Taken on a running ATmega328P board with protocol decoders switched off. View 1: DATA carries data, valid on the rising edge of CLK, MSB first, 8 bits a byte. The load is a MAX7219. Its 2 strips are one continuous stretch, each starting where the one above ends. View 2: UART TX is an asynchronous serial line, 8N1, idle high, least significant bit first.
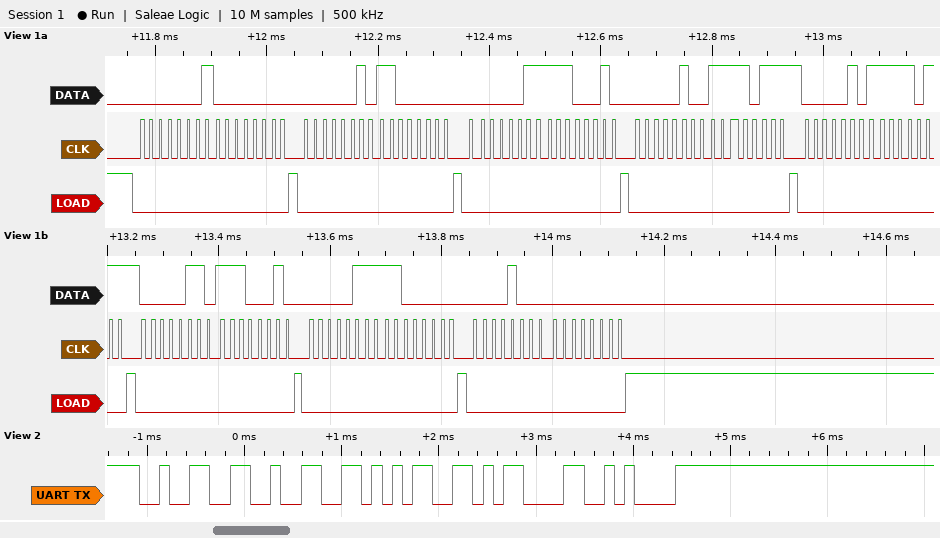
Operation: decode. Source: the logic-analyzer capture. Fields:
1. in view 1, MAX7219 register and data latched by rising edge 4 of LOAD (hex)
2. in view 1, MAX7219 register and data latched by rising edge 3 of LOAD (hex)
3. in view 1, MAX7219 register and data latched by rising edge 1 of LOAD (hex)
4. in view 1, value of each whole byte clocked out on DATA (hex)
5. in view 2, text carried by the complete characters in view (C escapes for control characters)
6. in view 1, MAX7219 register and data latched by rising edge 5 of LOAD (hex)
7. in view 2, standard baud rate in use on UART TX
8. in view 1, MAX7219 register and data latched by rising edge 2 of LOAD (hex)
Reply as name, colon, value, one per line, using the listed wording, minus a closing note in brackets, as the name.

in view 1, MAX7219 register and data latched by rising edge 4 of LOAD: register 0x4, data 0xF7
in view 1, MAX7219 register and data latched by rising edge 3 of LOAD: register 0x3, data 0xE2
in view 1, MAX7219 register and data latched by rising edge 1 of LOAD: register 0x1, data 0x00
in view 1, value of each whole byte clocked out on DATA: 01 00 02 C0 03 E2 04 F7 05 F7 06 E2 07 C0 08 00
in view 2, text carried by the complete characters in view: "225\r\n"
in view 1, MAX7219 register and data latched by rising edge 5 of LOAD: register 0x5, data 0xF7
in view 2, standard baud rate in use on UART TX: 9600 baud
in view 1, MAX7219 register and data latched by rising edge 2 of LOAD: register 0x2, data 0xC0
